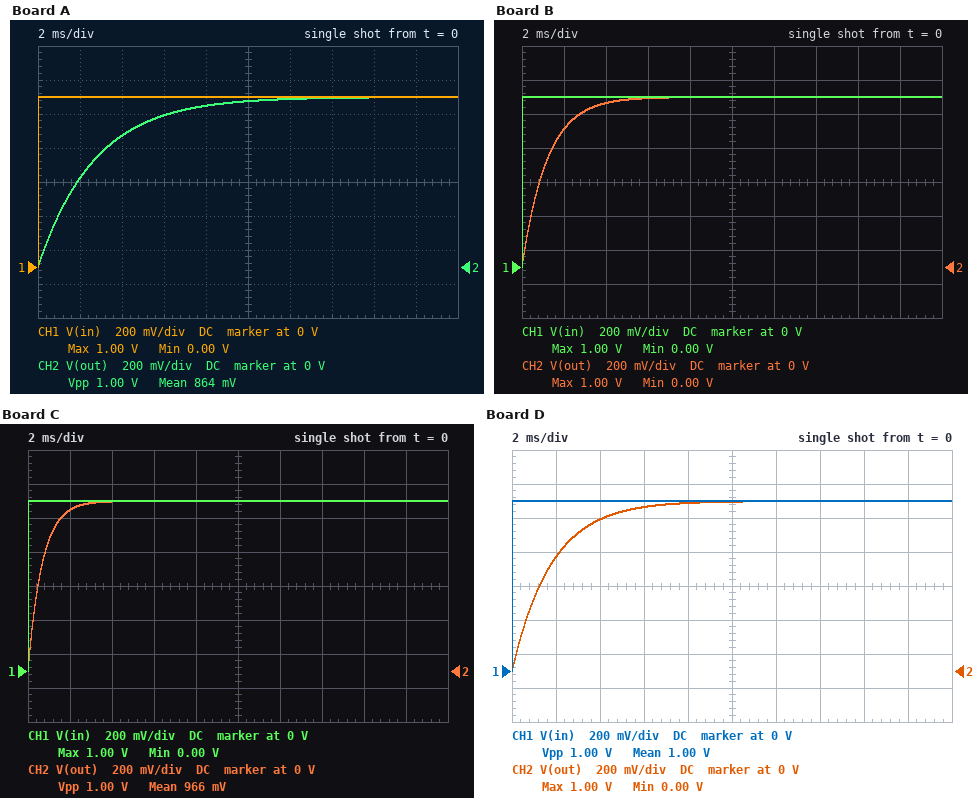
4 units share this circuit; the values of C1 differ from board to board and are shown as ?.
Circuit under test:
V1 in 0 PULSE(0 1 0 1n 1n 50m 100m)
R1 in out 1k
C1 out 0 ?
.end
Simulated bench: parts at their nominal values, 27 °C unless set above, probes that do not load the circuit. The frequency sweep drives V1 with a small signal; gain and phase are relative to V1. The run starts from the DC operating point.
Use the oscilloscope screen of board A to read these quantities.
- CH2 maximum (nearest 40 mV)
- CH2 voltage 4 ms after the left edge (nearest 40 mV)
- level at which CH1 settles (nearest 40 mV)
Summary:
1.00 V
760 mV
1.00 V
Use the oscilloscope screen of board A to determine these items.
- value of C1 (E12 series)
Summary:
2.7 µF
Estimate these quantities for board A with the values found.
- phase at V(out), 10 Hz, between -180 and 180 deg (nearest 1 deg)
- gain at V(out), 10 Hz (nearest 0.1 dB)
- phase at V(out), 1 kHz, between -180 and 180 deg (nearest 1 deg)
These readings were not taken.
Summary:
-10 deg
-0.1 dB
-87 deg
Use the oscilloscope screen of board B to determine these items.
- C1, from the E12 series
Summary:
1.2 µF
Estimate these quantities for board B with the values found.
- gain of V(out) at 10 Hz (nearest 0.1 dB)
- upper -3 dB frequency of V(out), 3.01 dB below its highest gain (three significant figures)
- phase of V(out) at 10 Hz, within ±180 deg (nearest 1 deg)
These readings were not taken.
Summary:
0 dB
133 Hz
-4 deg
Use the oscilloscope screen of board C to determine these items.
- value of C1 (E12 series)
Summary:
680 nF
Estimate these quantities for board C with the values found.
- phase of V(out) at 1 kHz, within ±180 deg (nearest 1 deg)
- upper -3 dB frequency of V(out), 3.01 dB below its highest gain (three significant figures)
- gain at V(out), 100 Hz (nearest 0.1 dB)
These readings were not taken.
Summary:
-77 deg
234 Hz
-0.7 dB
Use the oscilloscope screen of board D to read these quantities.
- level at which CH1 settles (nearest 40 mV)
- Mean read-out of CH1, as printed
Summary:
1.00 V
1.00 V
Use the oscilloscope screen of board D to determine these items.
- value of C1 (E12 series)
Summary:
1.8 µF
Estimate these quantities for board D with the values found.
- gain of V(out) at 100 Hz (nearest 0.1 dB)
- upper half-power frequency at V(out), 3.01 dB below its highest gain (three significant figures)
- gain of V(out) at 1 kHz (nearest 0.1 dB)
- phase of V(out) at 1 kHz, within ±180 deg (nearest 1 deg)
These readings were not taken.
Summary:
-3.6 dB
88.4 Hz
-21.1 dB
-85 deg
